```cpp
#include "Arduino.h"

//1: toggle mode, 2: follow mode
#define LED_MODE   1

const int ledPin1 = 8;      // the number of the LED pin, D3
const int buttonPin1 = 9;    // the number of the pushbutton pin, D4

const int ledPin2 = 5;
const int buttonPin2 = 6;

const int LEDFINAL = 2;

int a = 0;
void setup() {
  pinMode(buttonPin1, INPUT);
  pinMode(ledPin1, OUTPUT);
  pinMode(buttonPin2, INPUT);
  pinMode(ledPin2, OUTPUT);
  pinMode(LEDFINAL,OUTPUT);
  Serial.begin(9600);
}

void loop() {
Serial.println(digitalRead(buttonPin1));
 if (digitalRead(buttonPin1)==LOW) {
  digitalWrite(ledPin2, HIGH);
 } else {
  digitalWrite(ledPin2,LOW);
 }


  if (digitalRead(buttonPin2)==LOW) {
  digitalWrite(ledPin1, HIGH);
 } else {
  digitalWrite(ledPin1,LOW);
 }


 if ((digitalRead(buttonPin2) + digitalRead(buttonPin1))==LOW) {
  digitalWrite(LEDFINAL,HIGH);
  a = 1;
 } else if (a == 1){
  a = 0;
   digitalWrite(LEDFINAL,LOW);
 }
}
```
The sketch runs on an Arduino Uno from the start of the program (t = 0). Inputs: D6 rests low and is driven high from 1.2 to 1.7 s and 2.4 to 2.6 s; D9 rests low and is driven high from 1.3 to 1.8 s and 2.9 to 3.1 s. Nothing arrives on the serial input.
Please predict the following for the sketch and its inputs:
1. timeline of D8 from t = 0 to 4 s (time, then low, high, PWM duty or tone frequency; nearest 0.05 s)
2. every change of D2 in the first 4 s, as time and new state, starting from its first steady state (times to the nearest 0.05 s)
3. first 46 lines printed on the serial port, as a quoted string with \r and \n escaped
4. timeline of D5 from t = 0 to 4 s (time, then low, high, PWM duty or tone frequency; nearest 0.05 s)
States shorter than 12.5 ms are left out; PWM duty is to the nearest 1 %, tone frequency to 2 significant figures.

0 s high; 1.2 s low; 1.7 s high; 2.4 s low; 2.6 s high
0 s high; 1.2 s low; 1.8 s high; 2.4 s low; 2.6 s high; 2.9 s low; 3.1 s high
"0\r\n0\r\n0\r\n0\r\n0\r\n0\r\n0\r\n0\r\n0\r\n0\r\n0\r\n0\r\n0\r\n0\r\n0\r\n0\r\n0\r\n0\r\n0\r\n0\r\n0\r\n0\r\n0\r\n0\r\n0\r\n0\r\n0\r\n0\r\n0\r\n0\r\n0\r\n0\r\n0\r\n0\r\n0\r\n0\r\n0\r\n0\r\n0\r\n0\r\n0\r\n0\r\n0\r\n0\r\n0\r\n0\r\n"
0 s high; 1.3 s low; 1.8 s high; 2.9 s low; 3.1 s high
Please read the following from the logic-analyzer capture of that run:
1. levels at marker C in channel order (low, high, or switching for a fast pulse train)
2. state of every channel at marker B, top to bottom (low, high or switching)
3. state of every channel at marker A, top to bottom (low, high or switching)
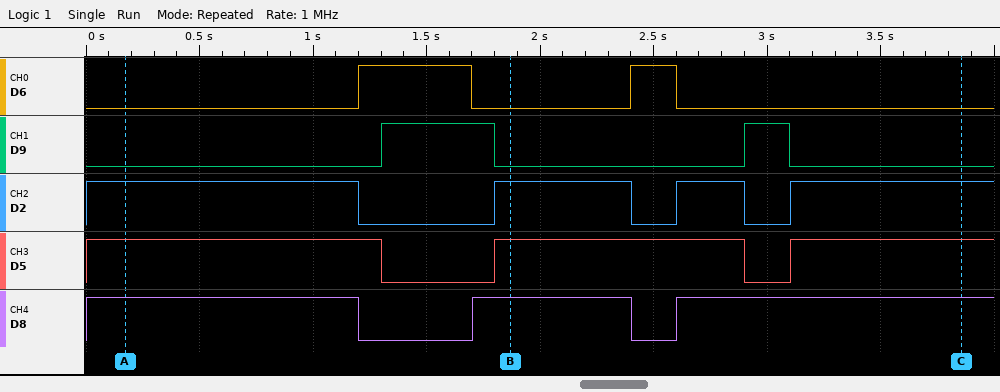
D6 low, D9 low, D2 high, D5 high, D8 high
D6 low, D9 low, D2 high, D5 high, D8 high
D6 low, D9 low, D2 high, D5 high, D8 high
